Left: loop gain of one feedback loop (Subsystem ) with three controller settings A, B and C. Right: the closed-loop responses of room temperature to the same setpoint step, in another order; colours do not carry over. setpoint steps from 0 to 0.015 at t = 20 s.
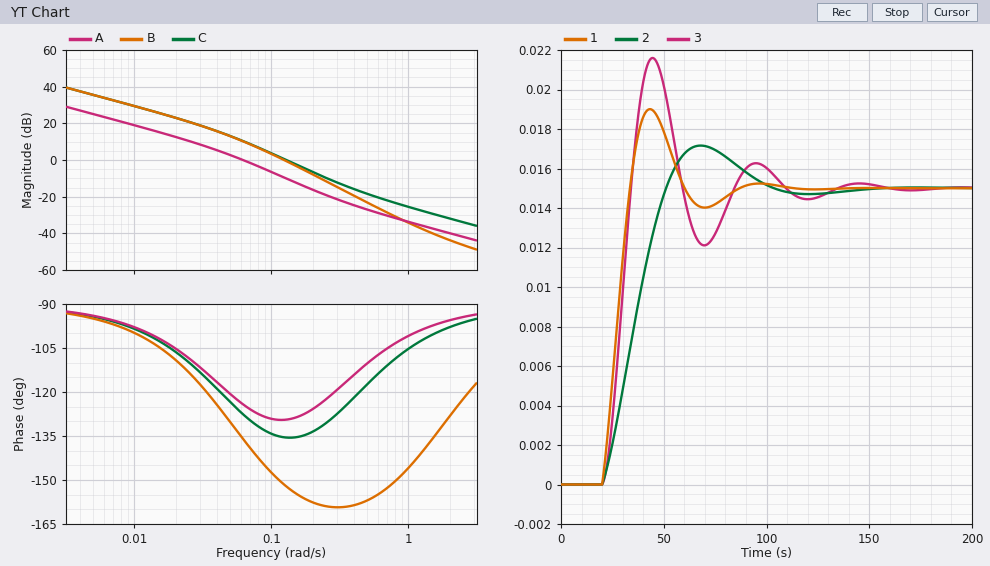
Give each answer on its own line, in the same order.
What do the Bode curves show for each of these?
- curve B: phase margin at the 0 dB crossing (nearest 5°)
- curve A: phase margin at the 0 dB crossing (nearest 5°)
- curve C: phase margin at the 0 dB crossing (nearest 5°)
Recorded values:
30°
55°
45°
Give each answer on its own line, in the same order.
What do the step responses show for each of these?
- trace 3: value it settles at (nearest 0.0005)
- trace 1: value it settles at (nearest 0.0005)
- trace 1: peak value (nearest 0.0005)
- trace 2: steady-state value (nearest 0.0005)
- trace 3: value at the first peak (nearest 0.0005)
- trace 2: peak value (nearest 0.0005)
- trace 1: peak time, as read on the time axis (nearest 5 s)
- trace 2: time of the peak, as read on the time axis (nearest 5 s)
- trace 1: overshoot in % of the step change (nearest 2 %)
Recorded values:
0.0150
0.0150
0.0190
0.0150
0.0215
0.0170
45 s
70 s
26 %
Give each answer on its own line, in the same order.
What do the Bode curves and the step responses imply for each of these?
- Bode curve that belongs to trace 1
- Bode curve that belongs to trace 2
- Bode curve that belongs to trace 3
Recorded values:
C
A
B
